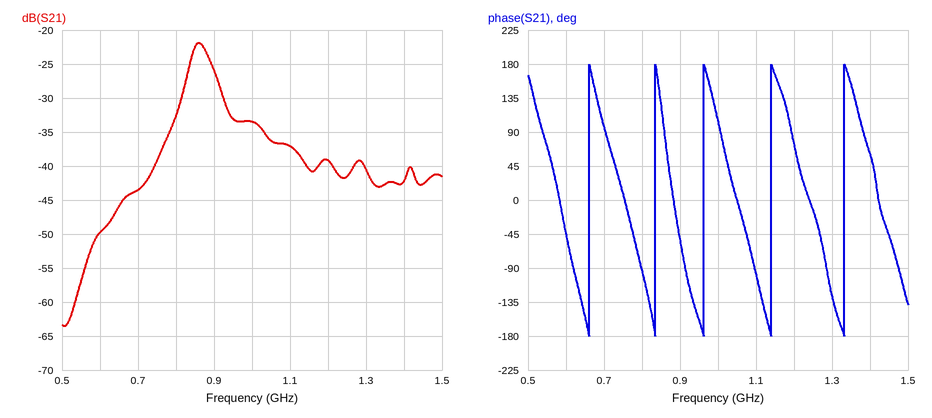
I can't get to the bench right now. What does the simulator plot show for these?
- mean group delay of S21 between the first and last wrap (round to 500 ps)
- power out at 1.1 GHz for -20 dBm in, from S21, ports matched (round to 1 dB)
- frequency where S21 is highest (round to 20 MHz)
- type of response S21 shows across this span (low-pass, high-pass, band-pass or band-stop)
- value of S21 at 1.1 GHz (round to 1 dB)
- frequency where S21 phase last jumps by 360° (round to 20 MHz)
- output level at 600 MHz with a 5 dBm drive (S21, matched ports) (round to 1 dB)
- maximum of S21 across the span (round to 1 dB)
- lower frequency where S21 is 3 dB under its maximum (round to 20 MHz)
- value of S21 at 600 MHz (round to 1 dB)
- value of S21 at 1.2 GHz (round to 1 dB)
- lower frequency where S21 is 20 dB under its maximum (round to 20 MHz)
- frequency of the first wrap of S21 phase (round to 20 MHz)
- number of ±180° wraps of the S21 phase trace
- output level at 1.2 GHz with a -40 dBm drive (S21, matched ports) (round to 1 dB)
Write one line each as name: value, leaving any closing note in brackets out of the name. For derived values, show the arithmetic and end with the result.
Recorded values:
mean group delay of S21 between the first and last wrap: 4 cycles / (1.34 GHz − 660 MHz) ≈ 5.88 ns, so 6.0 ns to the nearest 500 ps
power out at 1.1 GHz for -20 dBm in, from S21, ports matched: -20 dBm + (-37 dB) = -57 dBm
frequency where S21 is highest: 860 MHz
type of response S21 shows across this span: band-pass
value of S21 at 1.1 GHz: -37 dB
frequency where S21 phase last jumps by 360°: 1.34 GHz
output level at 600 MHz with a 5 dBm drive (S21, matched ports): 5 dBm + (-50 dB) = -45 dBm
maximum of S21 across the span: -22 dB
lower frequency where S21 is 3 dB under its maximum: 840 MHz
value of S21 at 600 MHz: -50 dB
value of S21 at 1.2 GHz: -39 dB
lower frequency where S21 is 20 dB under its maximum: 720 MHz
frequency of the first wrap of S21 phase: 660 MHz
number of ±180° wraps of the S21 phase trace: 5
output level at 1.2 GHz with a -40 dBm drive (S21, matched ports): -40 dBm + (-39 dB) = -79 dBm
